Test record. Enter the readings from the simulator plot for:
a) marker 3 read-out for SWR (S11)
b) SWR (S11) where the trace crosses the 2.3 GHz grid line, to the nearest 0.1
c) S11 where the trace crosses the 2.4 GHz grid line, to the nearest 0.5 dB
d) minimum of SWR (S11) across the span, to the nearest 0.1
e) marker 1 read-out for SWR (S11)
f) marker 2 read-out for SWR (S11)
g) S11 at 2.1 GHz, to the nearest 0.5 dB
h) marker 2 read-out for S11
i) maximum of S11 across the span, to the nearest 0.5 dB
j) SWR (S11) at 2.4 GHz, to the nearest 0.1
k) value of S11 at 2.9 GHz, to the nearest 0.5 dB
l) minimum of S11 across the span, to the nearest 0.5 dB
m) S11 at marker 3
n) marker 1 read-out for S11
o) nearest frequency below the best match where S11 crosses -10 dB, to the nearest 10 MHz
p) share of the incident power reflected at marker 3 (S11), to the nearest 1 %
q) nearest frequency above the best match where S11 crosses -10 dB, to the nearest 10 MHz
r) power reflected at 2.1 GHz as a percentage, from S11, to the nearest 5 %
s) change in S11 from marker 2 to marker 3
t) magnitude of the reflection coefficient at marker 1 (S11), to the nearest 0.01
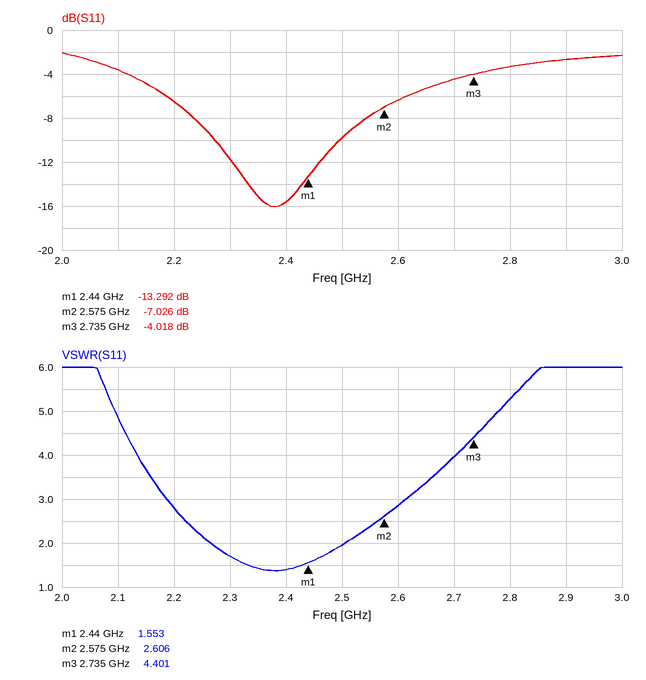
4.401
1.7
-15.5 dB
1.4
1.553
2.606
-3.5 dB
-7.026 dB
-2.0 dB
1.4
-2.5 dB
-16.0 dB
-4.018 dB
-13.292 dB
2.27 GHz
40 %
2.50 GHz
45 %
3.008 dB
0.22
